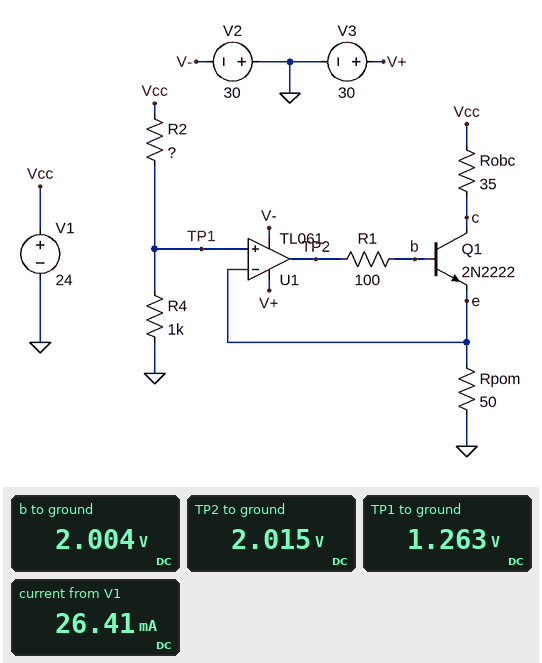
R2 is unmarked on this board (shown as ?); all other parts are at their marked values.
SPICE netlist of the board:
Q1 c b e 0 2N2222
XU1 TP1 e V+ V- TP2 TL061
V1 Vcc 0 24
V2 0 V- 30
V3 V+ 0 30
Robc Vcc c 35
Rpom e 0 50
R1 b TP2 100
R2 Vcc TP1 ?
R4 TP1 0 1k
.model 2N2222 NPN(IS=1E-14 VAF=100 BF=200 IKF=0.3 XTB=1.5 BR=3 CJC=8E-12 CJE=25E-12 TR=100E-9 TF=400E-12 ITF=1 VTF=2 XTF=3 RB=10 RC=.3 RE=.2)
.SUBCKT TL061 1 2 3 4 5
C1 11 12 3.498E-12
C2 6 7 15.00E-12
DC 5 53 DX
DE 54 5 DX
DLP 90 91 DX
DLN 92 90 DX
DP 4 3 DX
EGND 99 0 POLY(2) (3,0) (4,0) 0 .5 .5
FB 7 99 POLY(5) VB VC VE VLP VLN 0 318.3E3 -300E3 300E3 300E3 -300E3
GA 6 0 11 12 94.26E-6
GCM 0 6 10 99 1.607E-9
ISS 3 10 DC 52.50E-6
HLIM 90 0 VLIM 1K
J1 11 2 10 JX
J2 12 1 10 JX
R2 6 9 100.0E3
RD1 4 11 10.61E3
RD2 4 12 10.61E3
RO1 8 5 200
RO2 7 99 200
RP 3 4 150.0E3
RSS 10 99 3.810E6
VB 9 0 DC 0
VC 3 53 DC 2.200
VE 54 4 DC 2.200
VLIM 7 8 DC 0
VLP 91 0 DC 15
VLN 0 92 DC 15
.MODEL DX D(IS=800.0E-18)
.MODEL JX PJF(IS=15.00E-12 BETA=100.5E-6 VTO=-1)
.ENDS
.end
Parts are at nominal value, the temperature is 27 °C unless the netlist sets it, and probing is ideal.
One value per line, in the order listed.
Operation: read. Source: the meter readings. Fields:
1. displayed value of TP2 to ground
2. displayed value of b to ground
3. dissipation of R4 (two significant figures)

2.015 V
2.004 V
1.6 mW
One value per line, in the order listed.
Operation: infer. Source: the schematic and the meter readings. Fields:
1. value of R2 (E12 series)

18 kΩ
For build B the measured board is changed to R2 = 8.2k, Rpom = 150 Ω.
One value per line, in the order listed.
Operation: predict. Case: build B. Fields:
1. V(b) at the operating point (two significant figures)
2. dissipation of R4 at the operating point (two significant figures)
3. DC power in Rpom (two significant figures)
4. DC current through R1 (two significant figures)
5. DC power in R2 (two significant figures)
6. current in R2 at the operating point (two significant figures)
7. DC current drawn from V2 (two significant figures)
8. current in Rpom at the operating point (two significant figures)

3.3 V
6.8 mW
45 mW
76 µA
56 mW
2.6 mA
450 µA
17 mA
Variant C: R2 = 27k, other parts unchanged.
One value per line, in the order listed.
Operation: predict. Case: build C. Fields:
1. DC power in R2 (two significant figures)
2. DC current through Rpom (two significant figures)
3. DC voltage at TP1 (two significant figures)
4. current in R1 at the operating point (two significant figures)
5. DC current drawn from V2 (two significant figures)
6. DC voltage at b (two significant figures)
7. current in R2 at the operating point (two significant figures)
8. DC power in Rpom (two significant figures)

20 mW
17 mA
860 mV
73 µA
450 µA
1.6 V
860 µA
15 mW
